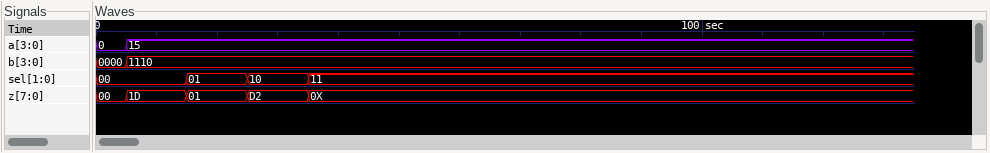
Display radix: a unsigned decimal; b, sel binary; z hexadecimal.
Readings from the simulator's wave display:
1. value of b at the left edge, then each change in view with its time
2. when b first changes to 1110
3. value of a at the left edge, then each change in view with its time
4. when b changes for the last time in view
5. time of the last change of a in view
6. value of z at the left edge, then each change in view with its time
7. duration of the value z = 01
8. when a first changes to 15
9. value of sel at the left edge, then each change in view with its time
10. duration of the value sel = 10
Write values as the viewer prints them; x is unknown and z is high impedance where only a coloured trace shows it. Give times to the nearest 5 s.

0000, 1110 at 5 s
5 s
0, 15 at 5 s
5 s
5 s
00, 1D at 5 s, 01 at 15 s, D2 at 25 s, 0X at 35 s
10 s
5 s
00, 01 at 15 s, 10 at 25 s, 11 at 35 s
10 s
